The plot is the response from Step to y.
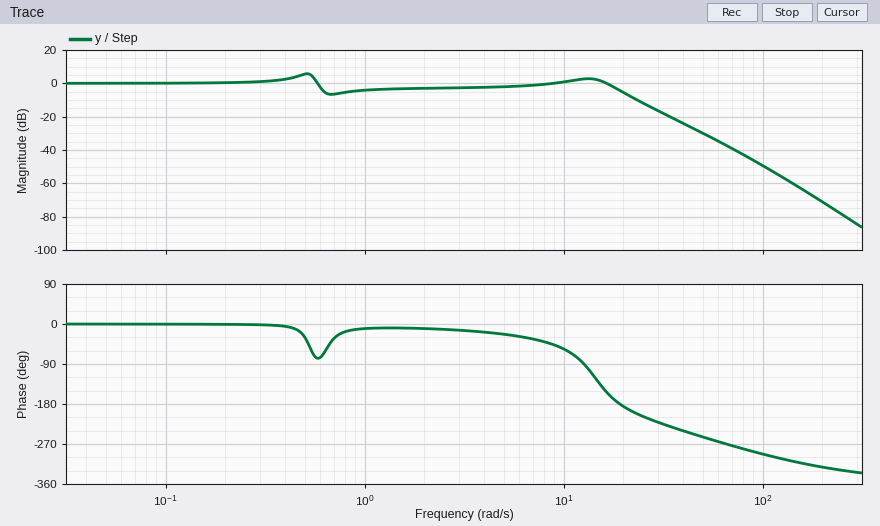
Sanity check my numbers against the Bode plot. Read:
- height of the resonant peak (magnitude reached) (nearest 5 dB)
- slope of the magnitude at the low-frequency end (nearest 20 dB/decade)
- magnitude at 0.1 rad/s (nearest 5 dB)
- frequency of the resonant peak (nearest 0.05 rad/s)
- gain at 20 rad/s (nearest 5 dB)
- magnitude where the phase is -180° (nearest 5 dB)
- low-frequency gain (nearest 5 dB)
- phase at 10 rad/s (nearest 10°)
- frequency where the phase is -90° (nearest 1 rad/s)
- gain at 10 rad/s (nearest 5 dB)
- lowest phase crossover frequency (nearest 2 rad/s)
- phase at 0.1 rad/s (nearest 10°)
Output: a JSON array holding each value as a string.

["5 dB", "0 dB/decade", "0 dB", "0.50 rad/s", "-5 dB", "-5 dB", "0 dB", "-60°", "13 rad/s", "0 dB", "20 rad/s", "0°"]
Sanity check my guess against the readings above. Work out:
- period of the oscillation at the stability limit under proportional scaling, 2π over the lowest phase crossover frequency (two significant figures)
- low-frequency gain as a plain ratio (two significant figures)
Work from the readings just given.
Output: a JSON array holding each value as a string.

["0.31 s", "1.0"]
